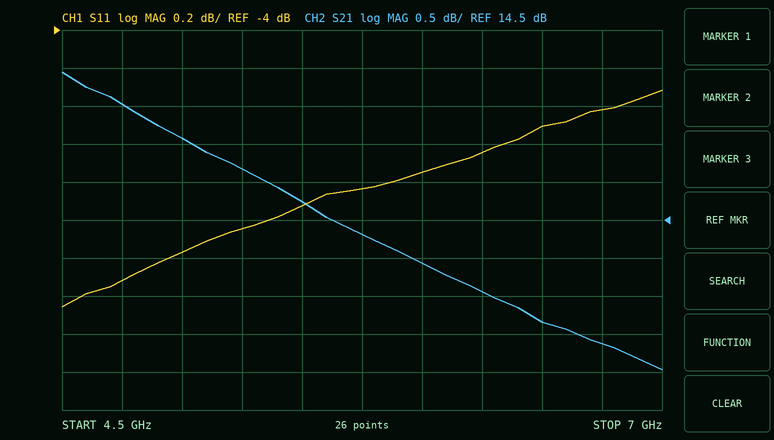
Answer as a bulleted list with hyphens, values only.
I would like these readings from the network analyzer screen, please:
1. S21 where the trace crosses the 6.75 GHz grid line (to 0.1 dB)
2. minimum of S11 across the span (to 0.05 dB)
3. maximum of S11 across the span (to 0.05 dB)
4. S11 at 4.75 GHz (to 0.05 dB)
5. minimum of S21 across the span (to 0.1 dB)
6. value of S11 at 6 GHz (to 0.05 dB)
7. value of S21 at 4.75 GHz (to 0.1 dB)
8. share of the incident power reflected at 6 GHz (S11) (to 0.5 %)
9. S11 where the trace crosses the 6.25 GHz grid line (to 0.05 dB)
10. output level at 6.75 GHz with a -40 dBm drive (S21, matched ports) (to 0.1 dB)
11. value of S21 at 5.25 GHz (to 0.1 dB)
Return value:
- 12.9 dB
- -5.45 dB
- -4.30 dB
- -5.30 dB
- 12.5 dB
- -4.75 dB
- 16.0 dB
- 33.5 %
- -4.65 dB
- -27.1 dBm
- 15.2 dB
